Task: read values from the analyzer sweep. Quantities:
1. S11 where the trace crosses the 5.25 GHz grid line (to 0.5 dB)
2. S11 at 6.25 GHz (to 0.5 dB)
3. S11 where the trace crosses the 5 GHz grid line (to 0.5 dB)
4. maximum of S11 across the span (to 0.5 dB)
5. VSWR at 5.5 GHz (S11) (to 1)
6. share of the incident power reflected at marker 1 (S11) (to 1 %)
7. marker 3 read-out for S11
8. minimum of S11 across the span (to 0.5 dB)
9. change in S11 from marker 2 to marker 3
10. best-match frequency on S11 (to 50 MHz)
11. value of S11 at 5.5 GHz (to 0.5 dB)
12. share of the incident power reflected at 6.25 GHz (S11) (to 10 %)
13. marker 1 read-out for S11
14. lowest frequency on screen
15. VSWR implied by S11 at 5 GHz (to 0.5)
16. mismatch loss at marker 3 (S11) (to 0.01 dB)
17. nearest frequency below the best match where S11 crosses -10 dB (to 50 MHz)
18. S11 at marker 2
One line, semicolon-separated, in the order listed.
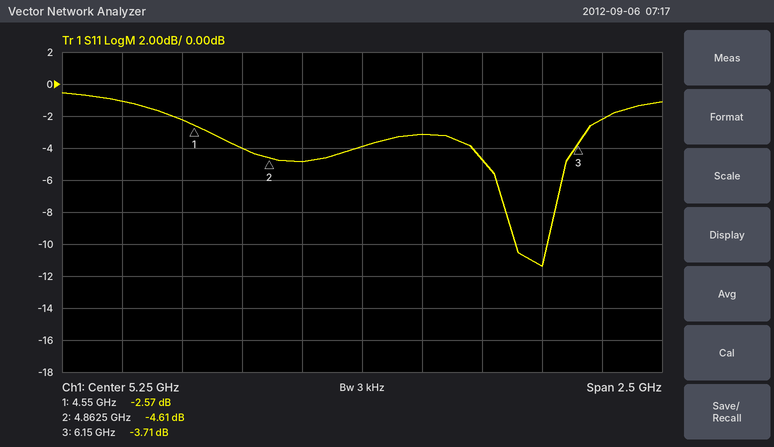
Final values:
-4.0 dB; -2.0 dB; -5.0 dB; -0.5 dB; 6; 55 %; -3.71 dB; -11.5 dB; 0.90 dB; 6.00 GHz; -3.0 dB; 60 %; -2.57 dB; 4 GHz; 3.5; 2.41 dB; 5.90 GHz; -4.61 dB
